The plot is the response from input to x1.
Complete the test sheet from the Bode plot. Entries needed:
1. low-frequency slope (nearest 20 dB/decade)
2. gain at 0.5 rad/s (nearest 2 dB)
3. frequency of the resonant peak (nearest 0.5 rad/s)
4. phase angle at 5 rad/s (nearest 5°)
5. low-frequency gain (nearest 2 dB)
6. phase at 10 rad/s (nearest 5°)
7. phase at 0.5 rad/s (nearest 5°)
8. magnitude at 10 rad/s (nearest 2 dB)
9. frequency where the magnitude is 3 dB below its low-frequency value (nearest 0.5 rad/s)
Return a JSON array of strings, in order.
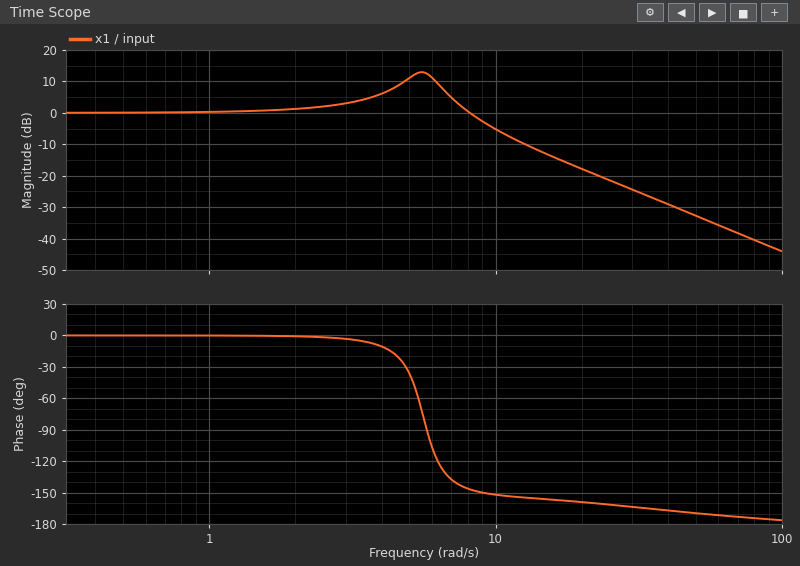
["0 dB/decade", "0 dB", "5.5 rad/s", "-35°", "0 dB", "-150°", "0°", "-6 dB", "9.0 rad/s"]
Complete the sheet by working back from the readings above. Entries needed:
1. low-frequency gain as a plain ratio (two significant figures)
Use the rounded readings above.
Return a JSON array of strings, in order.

["1.0"]
